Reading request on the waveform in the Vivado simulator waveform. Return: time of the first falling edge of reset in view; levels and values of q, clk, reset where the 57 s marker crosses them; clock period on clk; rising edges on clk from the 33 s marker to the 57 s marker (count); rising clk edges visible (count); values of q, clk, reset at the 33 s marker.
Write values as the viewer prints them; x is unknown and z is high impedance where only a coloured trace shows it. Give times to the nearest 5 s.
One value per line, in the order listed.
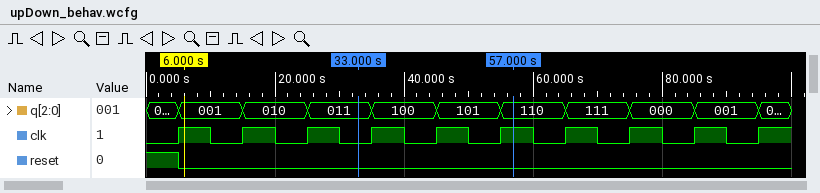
5 s
q=110, clk=1, reset=0
10 s
3
10
q=011, clk=0, reset=0
